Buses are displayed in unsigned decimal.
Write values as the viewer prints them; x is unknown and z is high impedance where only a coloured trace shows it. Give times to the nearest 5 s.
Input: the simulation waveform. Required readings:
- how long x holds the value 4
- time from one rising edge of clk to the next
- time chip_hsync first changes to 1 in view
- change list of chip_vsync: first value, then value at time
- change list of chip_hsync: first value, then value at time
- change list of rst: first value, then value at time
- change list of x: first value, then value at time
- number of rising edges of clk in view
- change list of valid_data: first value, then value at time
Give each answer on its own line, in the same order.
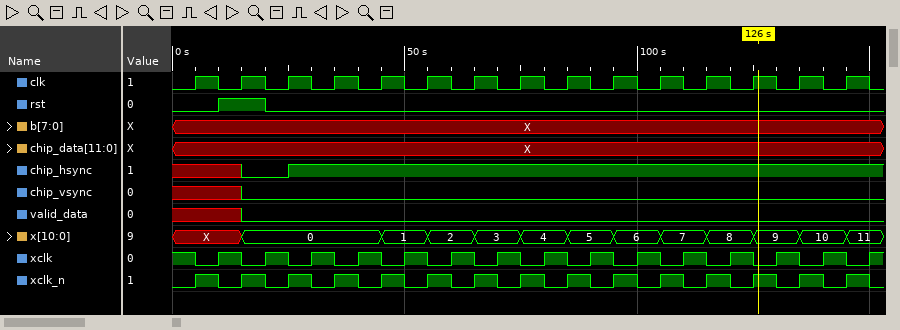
10 s
10 s
25 s
x, 0 at 15 s
x, 0 at 15 s, 1 at 25 s
0, 1 at 10 s, 0 at 20 s
X, 0 at 15 s, 1 at 45 s, 2 at 55 s, 3 at 65 s, 4 at 75 s, 5 at 85 s, 6 at 95 s, 7 at 105 s, 8 at 115 s, 9 at 125 s, 10 at 135 s, 11 at 145 s
15
x, 0 at 15 s
